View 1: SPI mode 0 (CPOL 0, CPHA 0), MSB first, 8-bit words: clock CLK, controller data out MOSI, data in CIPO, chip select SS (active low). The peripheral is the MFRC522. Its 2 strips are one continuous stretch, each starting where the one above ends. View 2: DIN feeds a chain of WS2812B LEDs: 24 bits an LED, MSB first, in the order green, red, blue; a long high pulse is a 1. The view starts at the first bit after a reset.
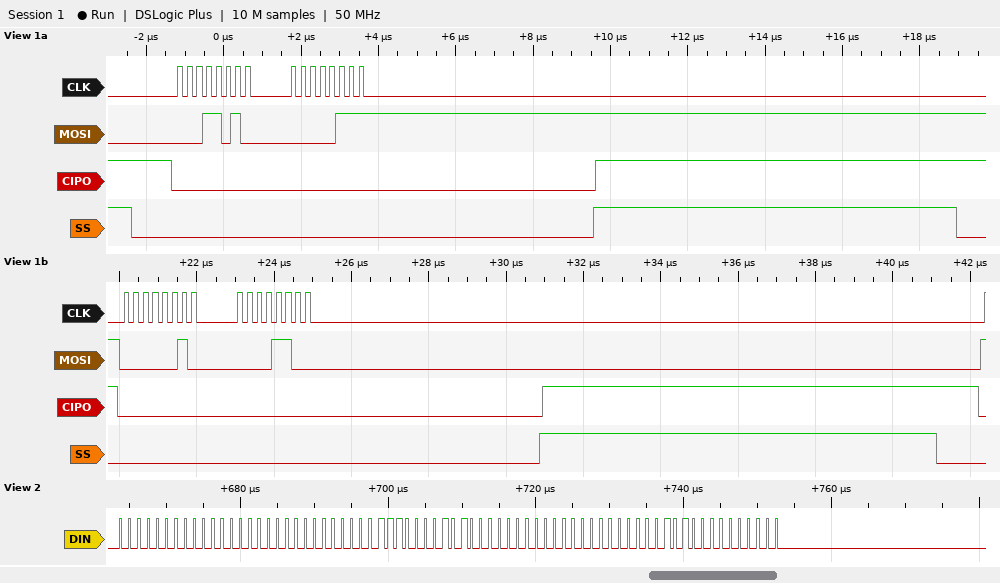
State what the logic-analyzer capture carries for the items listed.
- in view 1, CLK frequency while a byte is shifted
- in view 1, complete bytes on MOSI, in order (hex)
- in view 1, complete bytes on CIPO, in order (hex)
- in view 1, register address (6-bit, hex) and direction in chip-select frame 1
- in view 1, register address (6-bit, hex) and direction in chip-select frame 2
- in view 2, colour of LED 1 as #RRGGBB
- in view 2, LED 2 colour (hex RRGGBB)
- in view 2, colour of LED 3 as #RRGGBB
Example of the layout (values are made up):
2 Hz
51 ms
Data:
4 MHz
1A 07 02 0C
00 00 00 00
0x0D write
0x01 write
#000000
#140E00
#140000
